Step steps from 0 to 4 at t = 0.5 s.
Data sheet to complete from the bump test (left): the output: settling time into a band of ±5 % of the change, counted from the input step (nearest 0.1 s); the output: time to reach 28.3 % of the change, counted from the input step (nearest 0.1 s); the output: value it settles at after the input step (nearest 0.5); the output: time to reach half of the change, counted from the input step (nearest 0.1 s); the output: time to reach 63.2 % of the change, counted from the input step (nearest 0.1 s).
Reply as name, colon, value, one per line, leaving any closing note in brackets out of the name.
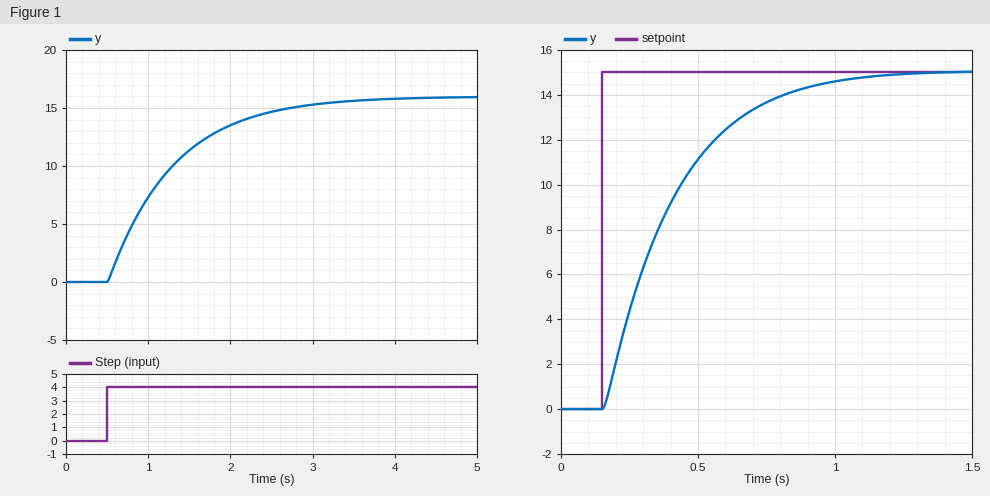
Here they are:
the output: settling time into a band of ±5 % of the change, counted from the input step: 2.4 s
the output: time to reach 28.3 % of the change, counted from the input step: 0.3 s
the output: value it settles at after the input step: 16.0
the output: time to reach half of the change, counted from the input step: 0.6 s
the output: time to reach 63.2 % of the change, counted from the input step: 0.8 s
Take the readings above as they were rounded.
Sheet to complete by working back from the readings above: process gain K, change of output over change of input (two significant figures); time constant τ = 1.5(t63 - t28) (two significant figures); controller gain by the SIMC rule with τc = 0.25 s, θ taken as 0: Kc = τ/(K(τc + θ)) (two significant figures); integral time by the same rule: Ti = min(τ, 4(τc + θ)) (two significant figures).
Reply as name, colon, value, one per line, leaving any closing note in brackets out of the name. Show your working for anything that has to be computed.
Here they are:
process gain K, change of output over change of input: (16 - 0) / 4 = 4.0
time constant τ = 1.5(t63 - t28): 1.5 × (0.8 - 0.3) = 0.75 s
controller gain by the SIMC rule with τc = 0.25 s, θ taken as 0: Kc = τ/(K(τc + θ)): 0.75 / (4 × (0.25 + 0)) = 0.75
integral time by the same rule: Ti = min(τ, 4(τc + θ)): min(0.75, 4 × (0.25 + 0)) = 0.75 s
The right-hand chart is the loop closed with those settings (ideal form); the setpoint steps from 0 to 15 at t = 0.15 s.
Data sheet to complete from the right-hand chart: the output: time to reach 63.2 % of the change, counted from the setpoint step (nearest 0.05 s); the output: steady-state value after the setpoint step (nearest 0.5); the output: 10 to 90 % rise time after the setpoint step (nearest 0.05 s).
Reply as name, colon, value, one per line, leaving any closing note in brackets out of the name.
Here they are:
the output: time to reach 63.2 % of the change, counted from the setpoint step: 0.25 s
the output: steady-state value after the setpoint step: 15.0
the output: 10 to 90 % rise time after the setpoint step: 0.55 s
